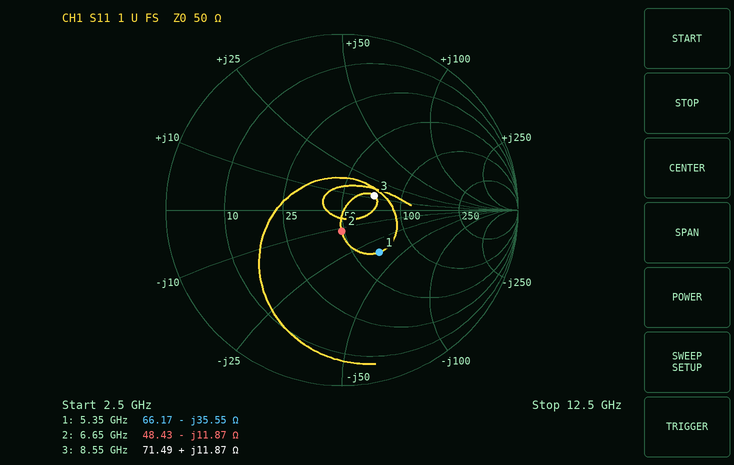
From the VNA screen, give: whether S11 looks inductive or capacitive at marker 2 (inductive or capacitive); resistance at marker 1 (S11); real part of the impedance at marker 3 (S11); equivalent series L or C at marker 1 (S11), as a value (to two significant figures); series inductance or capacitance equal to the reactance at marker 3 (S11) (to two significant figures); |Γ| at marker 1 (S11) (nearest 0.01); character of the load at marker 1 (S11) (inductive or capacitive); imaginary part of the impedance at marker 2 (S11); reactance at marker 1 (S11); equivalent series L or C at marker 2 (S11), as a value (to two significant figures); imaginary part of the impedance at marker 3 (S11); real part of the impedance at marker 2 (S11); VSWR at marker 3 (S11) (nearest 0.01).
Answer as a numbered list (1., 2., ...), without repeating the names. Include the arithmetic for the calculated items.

1. capacitive
2. 66.17 Ω
3. 71.49 Ω
4. C = 1/(2π × 5.35 GHz × 35.55 Ω) ≈ 837 fF, so 840 fF to two significant figures
5. L = 11.87 Ω/(2π × 8.55 GHz) ≈ 221 pH, so 220 pH to two significant figures
6. 0.32
7. capacitive
8. -11.87 Ω
9. -35.55 Ω
10. C = 1/(2π × 6.65 GHz × 11.87 Ω) ≈ 2.0 pF
11. +11.87 Ω
12. 48.43 Ω
13. 1.50
